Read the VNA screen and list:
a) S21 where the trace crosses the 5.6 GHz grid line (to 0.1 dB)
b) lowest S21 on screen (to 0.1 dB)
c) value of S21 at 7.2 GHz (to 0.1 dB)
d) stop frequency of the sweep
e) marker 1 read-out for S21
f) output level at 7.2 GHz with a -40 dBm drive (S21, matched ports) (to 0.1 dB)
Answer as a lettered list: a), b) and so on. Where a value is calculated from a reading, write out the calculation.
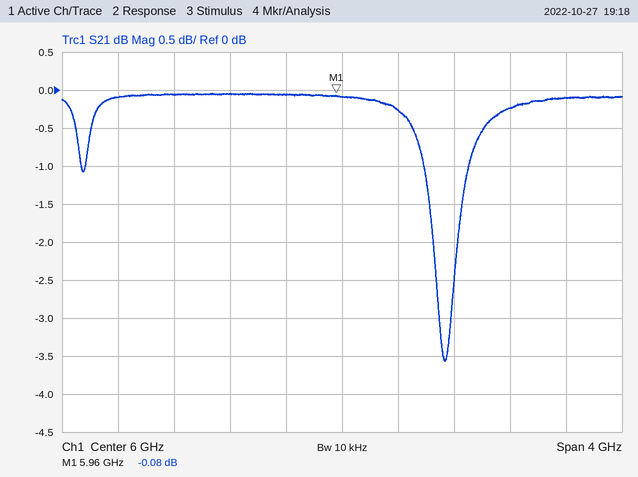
a) -0.1 dB
b) -3.6 dB
c) -0.2 dB
d) 8 GHz
e) -0.08 dB
f) -40 dBm + (-0.2 dB) = -40.2 dBm
